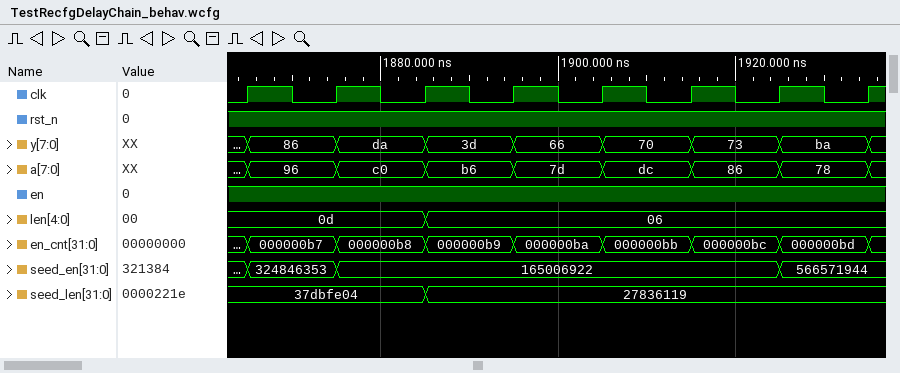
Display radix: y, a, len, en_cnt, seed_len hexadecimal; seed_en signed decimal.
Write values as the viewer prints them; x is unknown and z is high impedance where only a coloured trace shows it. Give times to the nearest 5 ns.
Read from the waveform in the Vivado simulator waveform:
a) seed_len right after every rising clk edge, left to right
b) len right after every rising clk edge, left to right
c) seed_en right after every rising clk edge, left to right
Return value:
37dbfe04, 37dbfe04, 27836119, 27836119, 27836119, 27836119, 27836119, 27836119
0d, 0d, 06, 06, 06, 06, 06, 06
324846353, 165006922, 165006922, 165006922, 165006922, 165006922, 566571944, 566571944
